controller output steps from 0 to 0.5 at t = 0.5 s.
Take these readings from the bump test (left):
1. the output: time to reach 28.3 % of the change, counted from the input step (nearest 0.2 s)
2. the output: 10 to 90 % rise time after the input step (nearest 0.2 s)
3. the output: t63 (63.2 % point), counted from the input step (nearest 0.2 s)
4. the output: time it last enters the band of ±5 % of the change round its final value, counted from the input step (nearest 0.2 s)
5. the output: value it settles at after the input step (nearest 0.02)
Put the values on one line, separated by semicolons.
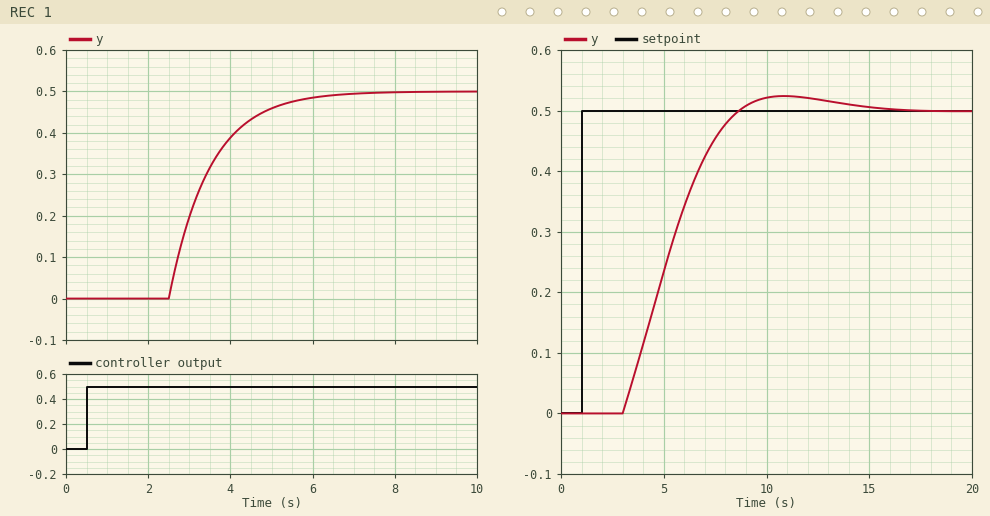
2.4 s; 2.2 s; 3.0 s; 5.0 s; 0.50
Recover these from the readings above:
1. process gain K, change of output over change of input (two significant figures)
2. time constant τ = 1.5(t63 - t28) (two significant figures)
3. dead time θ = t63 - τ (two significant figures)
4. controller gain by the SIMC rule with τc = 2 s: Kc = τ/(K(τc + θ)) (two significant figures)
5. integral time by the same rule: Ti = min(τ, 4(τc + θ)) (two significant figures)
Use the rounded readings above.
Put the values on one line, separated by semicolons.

1.0; 0.90 s; 2.1 s; 0.22; 0.90 s
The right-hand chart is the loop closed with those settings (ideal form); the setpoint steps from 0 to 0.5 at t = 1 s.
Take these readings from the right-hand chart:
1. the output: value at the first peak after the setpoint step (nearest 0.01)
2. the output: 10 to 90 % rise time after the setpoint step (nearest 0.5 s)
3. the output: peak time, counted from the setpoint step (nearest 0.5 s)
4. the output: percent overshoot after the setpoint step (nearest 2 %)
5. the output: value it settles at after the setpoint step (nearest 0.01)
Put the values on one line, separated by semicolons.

0.52; 4.0 s; 10.0 s; 4 %; 0.50
